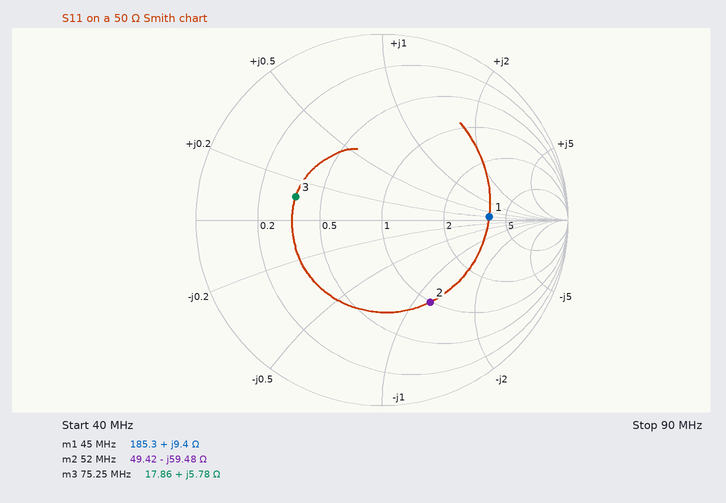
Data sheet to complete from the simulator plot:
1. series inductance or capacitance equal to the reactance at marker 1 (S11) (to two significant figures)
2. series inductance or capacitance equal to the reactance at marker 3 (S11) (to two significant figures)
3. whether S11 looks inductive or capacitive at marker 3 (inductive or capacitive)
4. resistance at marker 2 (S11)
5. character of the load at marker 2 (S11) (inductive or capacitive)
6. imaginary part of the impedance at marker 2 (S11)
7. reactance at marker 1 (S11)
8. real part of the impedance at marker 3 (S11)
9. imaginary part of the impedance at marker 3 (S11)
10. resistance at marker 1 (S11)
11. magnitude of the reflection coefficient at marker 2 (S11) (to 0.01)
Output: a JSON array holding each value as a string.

["33 nH", "12 nH", "inductive", "49.42 Ω", "capacitive", "-59.48 Ω", "+9.4 Ω", "17.86 Ω", "+5.78 Ω", "185.3 Ω", "0.51"]
